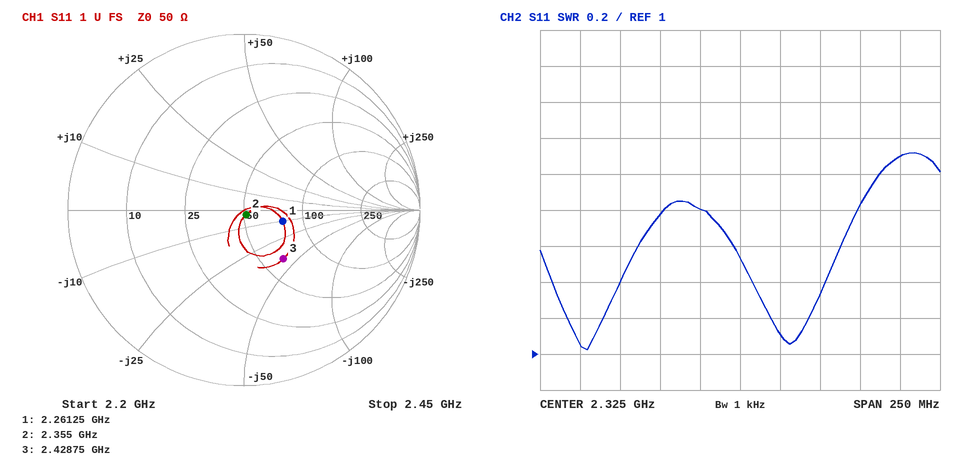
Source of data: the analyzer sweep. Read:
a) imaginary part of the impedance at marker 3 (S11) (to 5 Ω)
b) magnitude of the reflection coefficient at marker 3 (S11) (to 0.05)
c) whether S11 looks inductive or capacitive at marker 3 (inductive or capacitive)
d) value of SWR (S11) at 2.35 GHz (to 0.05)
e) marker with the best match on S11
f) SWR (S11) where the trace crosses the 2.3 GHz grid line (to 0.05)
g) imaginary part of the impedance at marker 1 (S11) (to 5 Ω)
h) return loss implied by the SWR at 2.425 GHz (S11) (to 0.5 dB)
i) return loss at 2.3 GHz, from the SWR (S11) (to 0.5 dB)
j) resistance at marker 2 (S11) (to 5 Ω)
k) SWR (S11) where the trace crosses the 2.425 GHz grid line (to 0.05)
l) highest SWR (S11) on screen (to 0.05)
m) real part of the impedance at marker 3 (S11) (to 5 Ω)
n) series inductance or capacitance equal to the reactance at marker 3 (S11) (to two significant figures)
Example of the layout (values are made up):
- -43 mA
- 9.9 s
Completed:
- -40 Ω
- 0.35
- capacitive
- 1.10
- marker 2
- 1.80
- -10 Ω
- 9.0 dB
- 11.0 dB
- 50 Ω
- 2.10
- 2.10
- 65 Ω
- 1.6 pF
